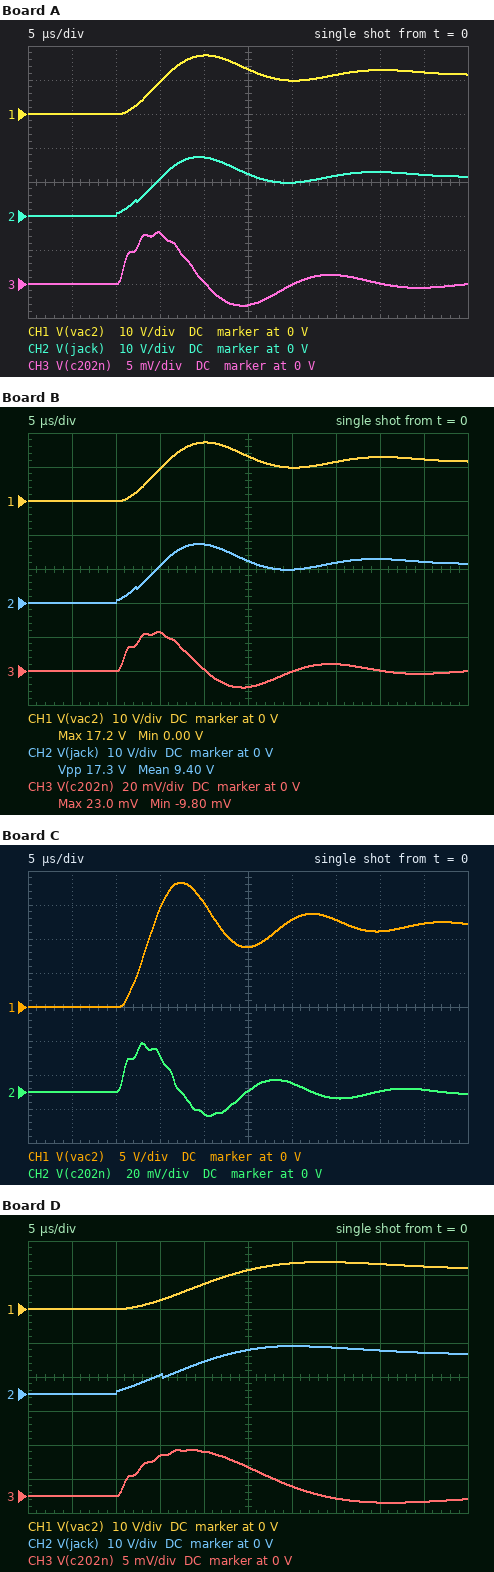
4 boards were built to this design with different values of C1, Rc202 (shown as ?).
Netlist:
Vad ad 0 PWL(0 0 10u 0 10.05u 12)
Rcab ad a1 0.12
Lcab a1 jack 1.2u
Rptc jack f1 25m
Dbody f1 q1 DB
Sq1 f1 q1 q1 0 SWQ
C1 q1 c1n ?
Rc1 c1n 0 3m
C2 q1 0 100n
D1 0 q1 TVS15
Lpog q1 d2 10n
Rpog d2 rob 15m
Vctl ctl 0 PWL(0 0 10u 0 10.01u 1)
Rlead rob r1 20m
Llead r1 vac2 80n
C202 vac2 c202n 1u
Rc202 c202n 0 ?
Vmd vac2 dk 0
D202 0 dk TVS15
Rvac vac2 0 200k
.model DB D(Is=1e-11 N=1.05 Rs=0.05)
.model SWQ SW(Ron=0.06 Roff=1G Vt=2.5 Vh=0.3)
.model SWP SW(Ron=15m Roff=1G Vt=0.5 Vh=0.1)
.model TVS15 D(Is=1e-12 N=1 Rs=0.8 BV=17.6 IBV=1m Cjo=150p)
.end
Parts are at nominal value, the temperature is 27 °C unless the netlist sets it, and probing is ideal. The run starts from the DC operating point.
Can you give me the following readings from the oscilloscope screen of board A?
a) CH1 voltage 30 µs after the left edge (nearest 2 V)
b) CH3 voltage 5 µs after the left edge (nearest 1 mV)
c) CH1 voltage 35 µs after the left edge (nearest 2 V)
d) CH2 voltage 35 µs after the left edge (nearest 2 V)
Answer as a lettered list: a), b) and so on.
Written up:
a) 10 V
b) 0 V
c) 12 V
d) 12 V
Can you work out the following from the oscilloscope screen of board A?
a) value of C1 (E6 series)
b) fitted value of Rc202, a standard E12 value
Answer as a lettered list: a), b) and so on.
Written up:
a) 6.8 µF
b) 2.7 mΩ
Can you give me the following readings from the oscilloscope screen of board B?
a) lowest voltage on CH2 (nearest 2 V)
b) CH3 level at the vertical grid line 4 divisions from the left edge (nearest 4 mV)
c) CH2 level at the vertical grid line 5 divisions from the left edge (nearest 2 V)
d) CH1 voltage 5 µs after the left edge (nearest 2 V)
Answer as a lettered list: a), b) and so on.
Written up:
a) 0 V
b) 0 V
c) 12 V
d) 0 V
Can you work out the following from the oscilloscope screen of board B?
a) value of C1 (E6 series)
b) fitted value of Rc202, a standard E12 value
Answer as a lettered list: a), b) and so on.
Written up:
a) 6.8 µF
b) 8.2 mΩ
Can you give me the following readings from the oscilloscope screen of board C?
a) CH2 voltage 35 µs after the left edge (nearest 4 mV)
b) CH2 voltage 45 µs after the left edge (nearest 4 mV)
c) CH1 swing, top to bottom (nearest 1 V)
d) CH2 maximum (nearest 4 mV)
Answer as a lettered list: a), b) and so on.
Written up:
a) -4 mV
b) 0 V
c) 18 V
d) 28 mV
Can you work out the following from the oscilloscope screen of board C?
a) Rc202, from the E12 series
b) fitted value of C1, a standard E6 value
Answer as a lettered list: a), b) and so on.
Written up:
a) 6.8 mΩ
b) 3.3 µF
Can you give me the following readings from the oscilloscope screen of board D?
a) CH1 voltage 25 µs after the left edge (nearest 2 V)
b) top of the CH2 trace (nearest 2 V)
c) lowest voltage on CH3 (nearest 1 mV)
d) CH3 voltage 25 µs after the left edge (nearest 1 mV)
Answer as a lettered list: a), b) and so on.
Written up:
a) 12 V
b) 14 V
c) -1 mV
d) 4 mV
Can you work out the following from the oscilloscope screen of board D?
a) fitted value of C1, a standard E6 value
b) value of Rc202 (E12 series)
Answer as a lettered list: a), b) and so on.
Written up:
a) 33 µF
b) 6.8 mΩ
